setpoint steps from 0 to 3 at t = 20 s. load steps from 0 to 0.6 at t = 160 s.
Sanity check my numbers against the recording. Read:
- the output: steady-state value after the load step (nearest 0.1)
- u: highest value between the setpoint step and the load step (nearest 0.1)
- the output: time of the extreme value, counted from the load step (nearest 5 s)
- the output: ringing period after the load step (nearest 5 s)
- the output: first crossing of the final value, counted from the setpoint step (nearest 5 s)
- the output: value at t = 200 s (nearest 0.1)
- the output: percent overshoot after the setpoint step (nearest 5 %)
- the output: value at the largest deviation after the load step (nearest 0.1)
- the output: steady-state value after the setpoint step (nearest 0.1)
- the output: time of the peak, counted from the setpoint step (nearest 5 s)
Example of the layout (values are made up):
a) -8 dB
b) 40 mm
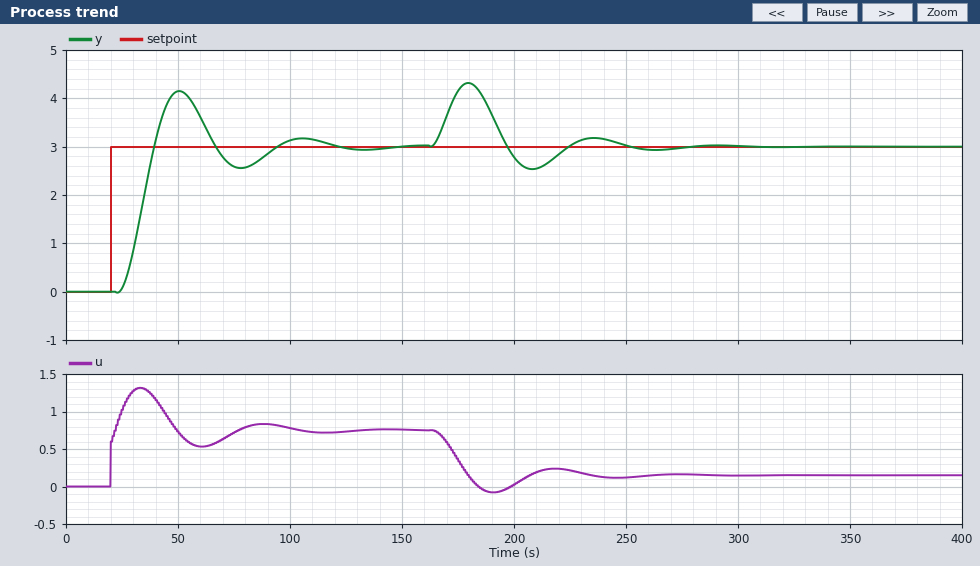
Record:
a) 3.0
b) 1.3
c) 20 s
d) 55 s
e) 20 s
f) 2.8
g) 40 %
h) 4.3
i) 3.0
j) 30 s
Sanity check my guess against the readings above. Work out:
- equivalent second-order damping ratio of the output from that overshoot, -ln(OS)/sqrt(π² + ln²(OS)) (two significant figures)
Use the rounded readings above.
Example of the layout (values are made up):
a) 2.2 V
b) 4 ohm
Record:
a) 0.28
